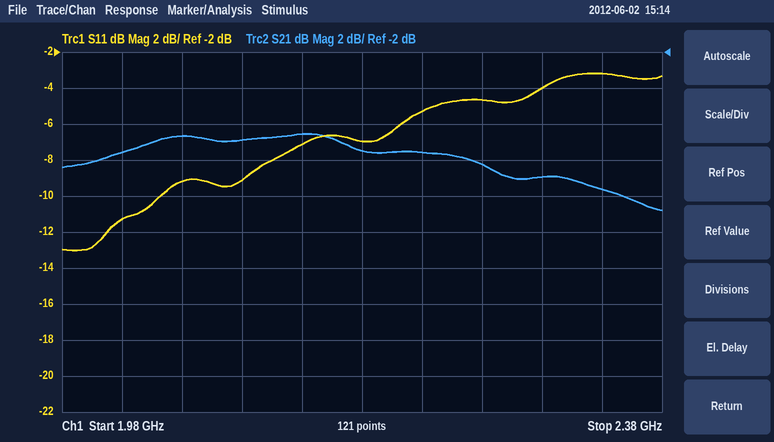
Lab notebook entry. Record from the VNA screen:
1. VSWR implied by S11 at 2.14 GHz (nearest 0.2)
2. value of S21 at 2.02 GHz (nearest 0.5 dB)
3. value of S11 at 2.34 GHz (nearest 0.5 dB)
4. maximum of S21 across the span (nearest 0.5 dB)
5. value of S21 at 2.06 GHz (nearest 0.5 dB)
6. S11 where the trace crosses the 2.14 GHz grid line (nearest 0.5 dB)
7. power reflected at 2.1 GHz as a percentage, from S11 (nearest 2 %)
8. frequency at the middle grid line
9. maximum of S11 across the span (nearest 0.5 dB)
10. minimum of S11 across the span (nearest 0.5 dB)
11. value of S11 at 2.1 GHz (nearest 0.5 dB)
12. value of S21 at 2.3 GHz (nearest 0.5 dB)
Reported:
2.6
-7.5 dB
-3.0 dB
-6.5 dB
-6.5 dB
-7.0 dB
12 %
2.18 GHz
-3.0 dB
-13.0 dB
-9.0 dB
-9.0 dB
